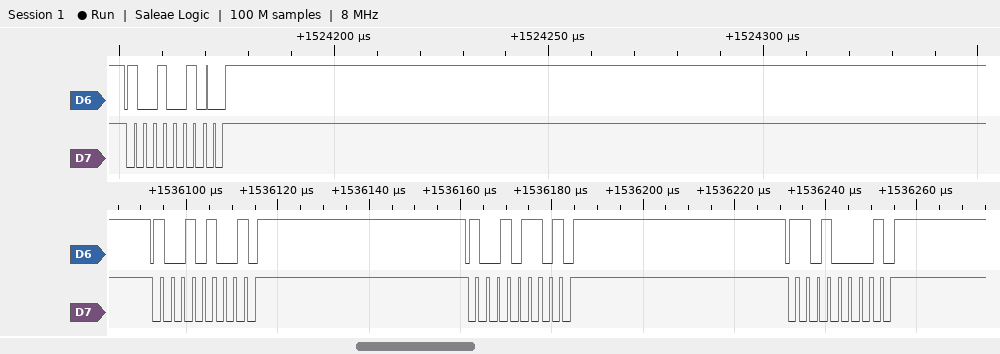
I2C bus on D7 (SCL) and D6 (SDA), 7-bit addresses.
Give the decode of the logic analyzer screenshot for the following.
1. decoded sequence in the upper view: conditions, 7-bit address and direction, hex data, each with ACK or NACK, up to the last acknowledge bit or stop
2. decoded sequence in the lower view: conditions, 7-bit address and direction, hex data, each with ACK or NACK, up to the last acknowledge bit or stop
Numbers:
start, address 49 write ACK, stop
start, address 4A write NACK, stop, start, address 4B write NACK, stop, start, address 68 write NACK, stop
